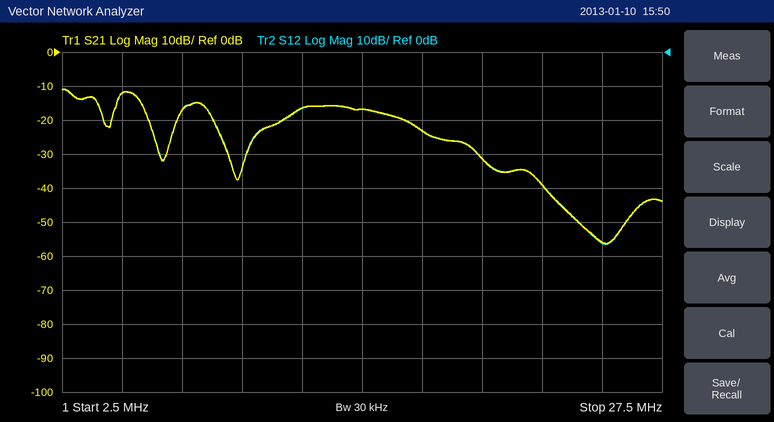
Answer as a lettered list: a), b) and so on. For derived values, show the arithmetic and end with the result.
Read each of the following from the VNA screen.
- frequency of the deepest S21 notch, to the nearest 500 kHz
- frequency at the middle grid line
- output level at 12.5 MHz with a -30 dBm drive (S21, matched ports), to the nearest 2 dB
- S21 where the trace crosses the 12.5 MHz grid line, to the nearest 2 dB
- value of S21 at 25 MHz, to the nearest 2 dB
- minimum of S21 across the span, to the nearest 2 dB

a) 25.0 MHz
b) 15 MHz
c) -30 dBm + (-16 dB) = -46 dBm
d) -16 dB
e) -56 dB
f) -56 dB
